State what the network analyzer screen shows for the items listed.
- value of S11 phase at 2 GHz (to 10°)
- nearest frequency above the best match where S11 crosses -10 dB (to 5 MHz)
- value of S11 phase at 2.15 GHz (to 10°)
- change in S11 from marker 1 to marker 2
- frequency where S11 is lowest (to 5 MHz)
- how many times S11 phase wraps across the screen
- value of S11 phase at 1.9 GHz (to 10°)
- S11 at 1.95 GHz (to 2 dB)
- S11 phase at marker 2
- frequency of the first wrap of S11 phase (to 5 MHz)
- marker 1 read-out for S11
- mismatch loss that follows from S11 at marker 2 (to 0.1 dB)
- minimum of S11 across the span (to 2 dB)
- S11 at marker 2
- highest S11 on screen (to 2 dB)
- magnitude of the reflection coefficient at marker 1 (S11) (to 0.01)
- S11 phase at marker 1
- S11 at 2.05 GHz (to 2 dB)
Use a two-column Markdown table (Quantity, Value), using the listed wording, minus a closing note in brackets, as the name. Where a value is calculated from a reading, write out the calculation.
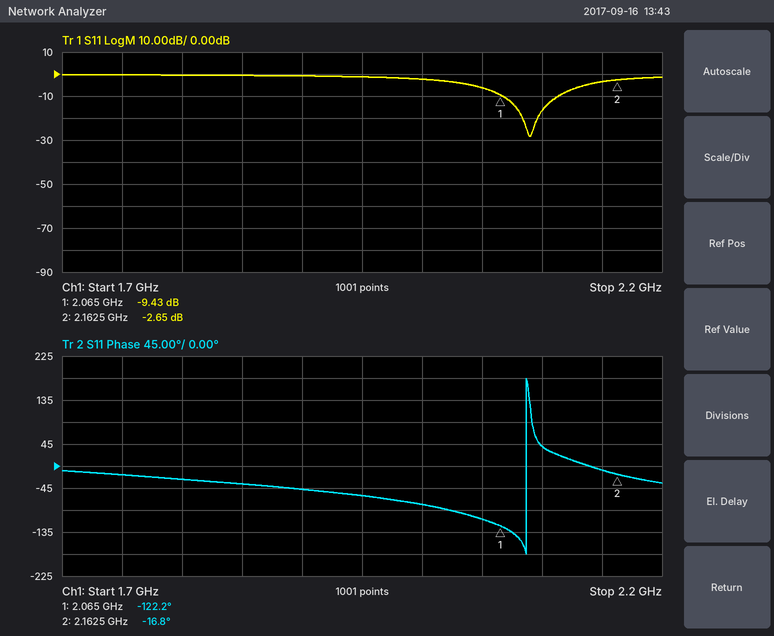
| Quantity | Value |
|---|---|
| value of S11 phase at 2 GHz | -80° |
| nearest frequency above the best match where S11 crosses -10 dB | 2.115 GHz |
| value of S11 phase at 2.15 GHz | -10° |
| change in S11 from marker 1 to marker 2 | -2.65 − (-9.43) = 6.78 dB |
| frequency where S11 is lowest | 2.090 GHz |
| how many times S11 phase wraps across the screen | 1 |
| value of S11 phase at 1.9 GHz | -50° |
| S11 at 1.95 GHz | -2 dB |
| S11 phase at marker 2 | -16.8° |
| frequency of the first wrap of S11 phase | 2.085 GHz |
| marker 1 read-out for S11 | -9.43 dB |
| mismatch loss that follows from S11 at marker 2 | −10 log10(1 − 10^(-2.65/10)) ≈ 3.4 dB |
| minimum of S11 across the span | -28 dB |
| S11 at marker 2 | -2.65 dB |
| highest S11 on screen | 0 dB |
| magnitude of the reflection coefficient at marker 1 (S11) | 10^(-9.43/20) ≈ 0.34 |
| S11 phase at marker 1 | -122.2° |
| S11 at 2.05 GHz | -6 dB |
